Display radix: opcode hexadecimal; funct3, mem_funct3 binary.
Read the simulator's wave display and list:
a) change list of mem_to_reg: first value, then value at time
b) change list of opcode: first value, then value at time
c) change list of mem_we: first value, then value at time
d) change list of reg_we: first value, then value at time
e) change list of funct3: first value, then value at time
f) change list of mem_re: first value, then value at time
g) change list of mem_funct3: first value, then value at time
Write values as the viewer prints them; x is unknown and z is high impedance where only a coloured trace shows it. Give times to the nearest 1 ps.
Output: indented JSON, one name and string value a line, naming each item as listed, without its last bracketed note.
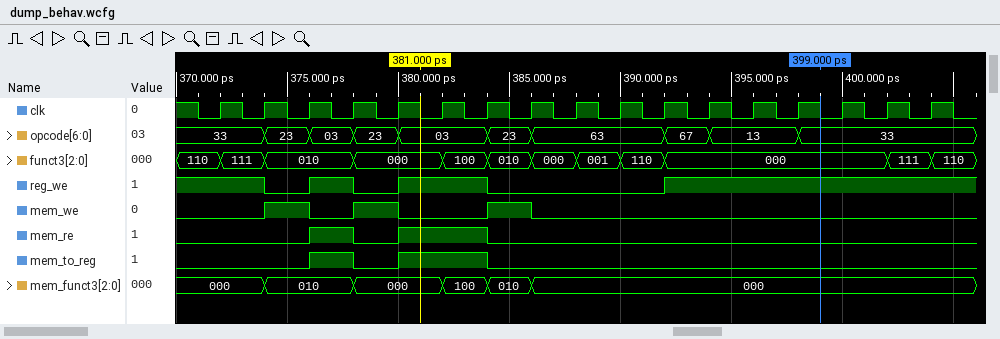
{
  "change list of mem_to_reg: first value, then value at time": "0, 1 at 376 ps, 0 at 378 ps, 1 at 380 ps, 0 at 384 ps",
  "change list of opcode: first value, then value at time": "33, 23 at 374 ps, 03 at 376 ps, 23 at 378 ps, 03 at 380 ps, 23 at 384 ps, 63 at 386 ps, 67 at 392 ps, 13 at 394 ps, 33 at 398 ps",
  "change list of mem_we: first value, then value at time": "0, 1 at 374 ps, 0 at 376 ps, 1 at 378 ps, 0 at 380 ps, 1 at 384 ps, 0 at 386 ps",
  "change list of reg_we: first value, then value at time": "1, 0 at 374 ps, 1 at 376 ps, 0 at 378 ps, 1 at 380 ps, 0 at 384 ps, 1 at 392 ps",
  "change list of funct3: first value, then value at time": "110, 111 at 372 ps, 010 at 374 ps, 000 at 378 ps, 100 at 382 ps, 010 at 384 ps, 000 at 386 ps, 001 at 388 ps, 110 at 390 ps, 000 at 392 ps, 111 at 402 ps, 110 at 404 ps",
  "change list of mem_re: first value, then value at time": "0, 1 at 376 ps, 0 at 378 ps, 1 at 380 ps, 0 at 384 ps",
  "change list of mem_funct3: first value, then value at time": "000, 010 at 374 ps, 000 at 378 ps, 100 at 382 ps, 010 at 384 ps, 000 at 386 ps"
}
